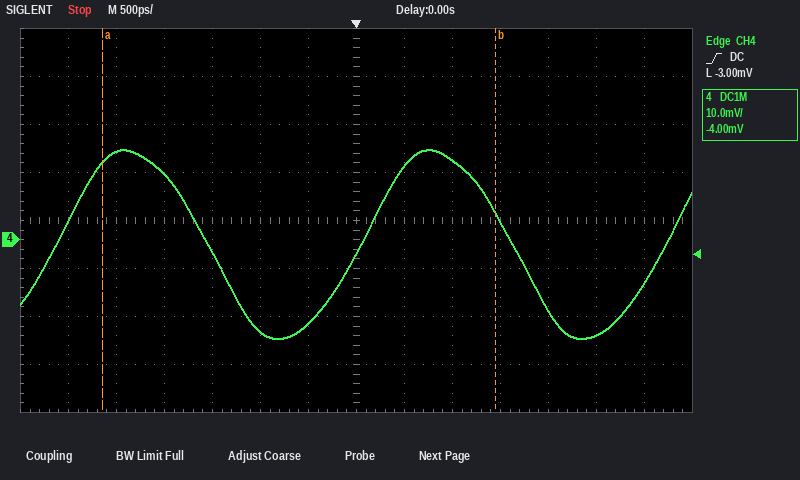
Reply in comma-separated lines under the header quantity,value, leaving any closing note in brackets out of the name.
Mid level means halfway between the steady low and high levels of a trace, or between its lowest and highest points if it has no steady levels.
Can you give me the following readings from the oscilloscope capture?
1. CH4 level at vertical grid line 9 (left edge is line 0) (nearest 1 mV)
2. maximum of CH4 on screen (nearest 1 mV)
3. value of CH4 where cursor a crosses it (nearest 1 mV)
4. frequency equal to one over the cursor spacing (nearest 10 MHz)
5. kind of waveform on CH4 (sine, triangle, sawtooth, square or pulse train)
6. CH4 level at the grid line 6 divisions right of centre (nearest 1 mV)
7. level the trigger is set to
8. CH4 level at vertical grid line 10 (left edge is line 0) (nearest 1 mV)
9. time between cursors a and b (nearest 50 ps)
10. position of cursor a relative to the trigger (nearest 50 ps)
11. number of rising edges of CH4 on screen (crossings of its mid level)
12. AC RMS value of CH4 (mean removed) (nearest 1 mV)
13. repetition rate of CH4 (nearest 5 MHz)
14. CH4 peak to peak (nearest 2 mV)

quantity,value
CH4 level at vertical grid line 9 (left edge is line 0),17 mV
maximum of CH4 on screen,19 mV
value of CH4 where cursor a crosses it,16 mV
frequency equal to one over the cursor spacing,240 MHz
kind of waveform on CH4,sine
CH4 level at the grid line 6 divisions right of centre,-9 mV
level the trigger is set to,-3.00 mV
CH4 level at vertical grid line 10 (left edge is line 0),4 mV
time between cursors a and b,4.10 ns
position of cursor a relative to the trigger,-2.65 ns
number of rising edges of CH4 on screen,3
AC RMS value of CH4 (mean removed),14 mV
repetition rate of CH4,315 MHz
CH4 peak to peak,40 mV
